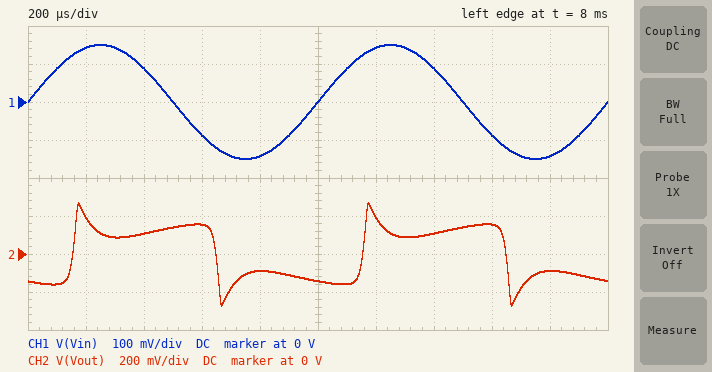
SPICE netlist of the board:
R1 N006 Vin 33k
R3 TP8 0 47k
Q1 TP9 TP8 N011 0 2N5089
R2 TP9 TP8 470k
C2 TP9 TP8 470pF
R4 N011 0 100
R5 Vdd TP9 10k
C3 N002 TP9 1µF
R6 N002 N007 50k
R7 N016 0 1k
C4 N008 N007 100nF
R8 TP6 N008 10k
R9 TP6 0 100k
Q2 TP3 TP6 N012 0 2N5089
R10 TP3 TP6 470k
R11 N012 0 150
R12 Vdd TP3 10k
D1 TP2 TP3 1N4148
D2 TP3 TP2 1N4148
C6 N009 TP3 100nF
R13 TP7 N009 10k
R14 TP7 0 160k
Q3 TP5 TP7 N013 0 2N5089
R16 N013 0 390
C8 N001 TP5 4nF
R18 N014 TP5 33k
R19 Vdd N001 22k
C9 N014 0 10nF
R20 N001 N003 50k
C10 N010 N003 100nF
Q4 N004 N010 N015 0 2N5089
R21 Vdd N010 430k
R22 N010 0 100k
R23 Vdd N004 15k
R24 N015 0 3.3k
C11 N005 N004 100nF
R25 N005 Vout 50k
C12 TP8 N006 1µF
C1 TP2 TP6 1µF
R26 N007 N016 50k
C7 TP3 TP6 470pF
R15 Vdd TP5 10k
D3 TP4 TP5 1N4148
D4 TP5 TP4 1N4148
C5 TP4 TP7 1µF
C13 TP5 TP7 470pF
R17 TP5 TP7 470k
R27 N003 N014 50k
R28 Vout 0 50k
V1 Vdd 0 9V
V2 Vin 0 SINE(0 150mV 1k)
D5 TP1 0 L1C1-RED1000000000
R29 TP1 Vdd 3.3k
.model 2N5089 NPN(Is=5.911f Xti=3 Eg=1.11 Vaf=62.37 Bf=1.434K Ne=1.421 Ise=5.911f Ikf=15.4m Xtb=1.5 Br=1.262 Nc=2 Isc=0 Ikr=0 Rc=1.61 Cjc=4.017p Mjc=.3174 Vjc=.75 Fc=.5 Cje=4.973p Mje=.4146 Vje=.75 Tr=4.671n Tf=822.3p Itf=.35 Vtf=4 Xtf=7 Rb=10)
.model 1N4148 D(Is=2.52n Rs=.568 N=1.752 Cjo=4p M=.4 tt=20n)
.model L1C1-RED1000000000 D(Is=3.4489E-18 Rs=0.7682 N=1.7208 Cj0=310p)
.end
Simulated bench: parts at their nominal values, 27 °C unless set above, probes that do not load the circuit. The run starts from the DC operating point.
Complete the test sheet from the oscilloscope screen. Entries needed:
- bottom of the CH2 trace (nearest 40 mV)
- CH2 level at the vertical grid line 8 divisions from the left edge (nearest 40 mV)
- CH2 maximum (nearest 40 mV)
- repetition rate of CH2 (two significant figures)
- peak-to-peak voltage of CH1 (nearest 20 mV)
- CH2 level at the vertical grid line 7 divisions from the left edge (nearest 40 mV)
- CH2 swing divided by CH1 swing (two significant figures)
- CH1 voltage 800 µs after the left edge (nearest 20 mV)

-280 mV
160 mV
280 mV
1.0 kHz
300 mV
120 mV
1.8
-140 mV
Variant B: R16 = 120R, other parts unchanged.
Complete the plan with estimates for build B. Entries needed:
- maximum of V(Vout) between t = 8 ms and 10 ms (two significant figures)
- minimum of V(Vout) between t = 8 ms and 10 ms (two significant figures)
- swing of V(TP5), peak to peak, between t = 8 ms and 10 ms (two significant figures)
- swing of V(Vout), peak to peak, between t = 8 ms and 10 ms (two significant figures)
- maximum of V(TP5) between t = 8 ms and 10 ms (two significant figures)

290 mV
-300 mV
830 mV
590 mV
3.6 V
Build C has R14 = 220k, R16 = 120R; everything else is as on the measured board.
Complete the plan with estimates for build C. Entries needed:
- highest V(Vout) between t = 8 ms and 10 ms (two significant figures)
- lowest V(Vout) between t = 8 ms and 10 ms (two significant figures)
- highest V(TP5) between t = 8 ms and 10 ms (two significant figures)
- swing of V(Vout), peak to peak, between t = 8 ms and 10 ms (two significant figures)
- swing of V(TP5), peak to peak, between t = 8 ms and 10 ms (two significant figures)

290 mV
-300 mV
3.1 V
590 mV
830 mV
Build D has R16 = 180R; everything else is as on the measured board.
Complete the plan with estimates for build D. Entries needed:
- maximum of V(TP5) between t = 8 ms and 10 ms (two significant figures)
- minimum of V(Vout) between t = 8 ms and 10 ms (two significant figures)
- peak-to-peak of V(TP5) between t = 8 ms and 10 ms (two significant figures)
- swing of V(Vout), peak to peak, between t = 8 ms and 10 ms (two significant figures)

3.8 V
-290 mV
820 mV
580 mV
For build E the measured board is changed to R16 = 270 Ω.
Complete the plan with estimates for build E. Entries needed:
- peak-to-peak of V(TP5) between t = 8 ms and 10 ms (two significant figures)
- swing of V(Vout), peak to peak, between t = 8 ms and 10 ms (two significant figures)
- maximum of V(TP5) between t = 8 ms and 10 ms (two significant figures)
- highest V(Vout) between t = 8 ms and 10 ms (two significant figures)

800 mV
560 mV
3.9 V
280 mV
